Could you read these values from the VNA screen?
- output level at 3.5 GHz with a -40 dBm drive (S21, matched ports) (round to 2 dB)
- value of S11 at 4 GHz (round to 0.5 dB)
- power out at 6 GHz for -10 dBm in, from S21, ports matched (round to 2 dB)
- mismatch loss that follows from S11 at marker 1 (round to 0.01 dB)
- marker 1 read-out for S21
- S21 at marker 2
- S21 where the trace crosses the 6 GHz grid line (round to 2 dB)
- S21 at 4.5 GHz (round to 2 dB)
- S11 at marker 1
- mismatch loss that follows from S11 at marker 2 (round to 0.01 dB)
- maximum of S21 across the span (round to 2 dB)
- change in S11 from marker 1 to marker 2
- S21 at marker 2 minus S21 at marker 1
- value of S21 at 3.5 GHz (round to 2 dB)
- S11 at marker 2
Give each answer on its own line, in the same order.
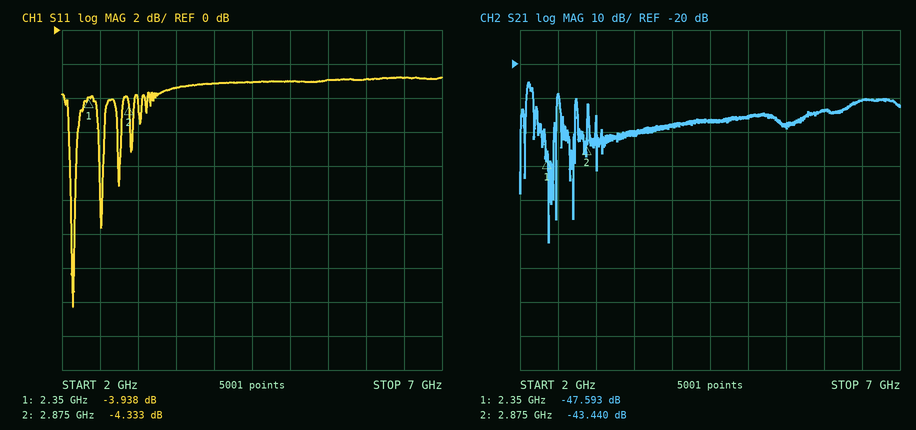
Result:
-80 dBm
-3.0 dB
-44 dBm
2.25 dB
-47.593 dB
-43.440 dB
-34 dB
-36 dB
-3.938 dB
2.00 dB
-26 dB
-0.395 dB
4.153 dB
-40 dB
-4.333 dB
